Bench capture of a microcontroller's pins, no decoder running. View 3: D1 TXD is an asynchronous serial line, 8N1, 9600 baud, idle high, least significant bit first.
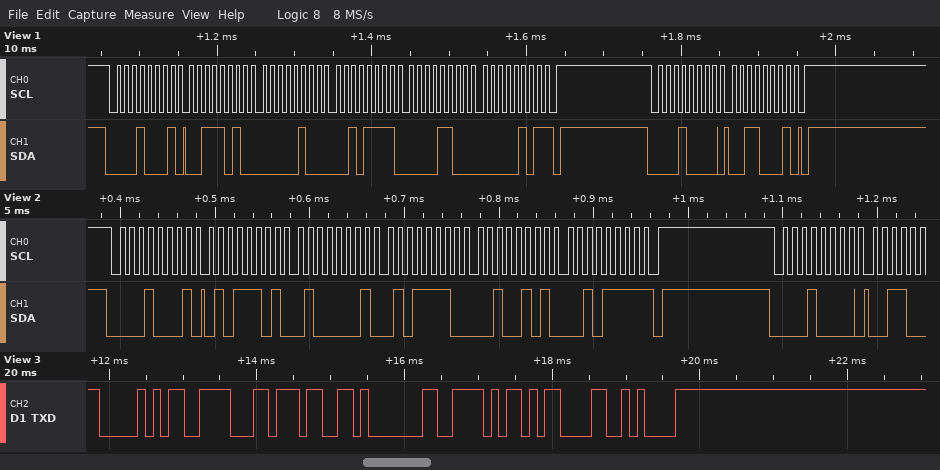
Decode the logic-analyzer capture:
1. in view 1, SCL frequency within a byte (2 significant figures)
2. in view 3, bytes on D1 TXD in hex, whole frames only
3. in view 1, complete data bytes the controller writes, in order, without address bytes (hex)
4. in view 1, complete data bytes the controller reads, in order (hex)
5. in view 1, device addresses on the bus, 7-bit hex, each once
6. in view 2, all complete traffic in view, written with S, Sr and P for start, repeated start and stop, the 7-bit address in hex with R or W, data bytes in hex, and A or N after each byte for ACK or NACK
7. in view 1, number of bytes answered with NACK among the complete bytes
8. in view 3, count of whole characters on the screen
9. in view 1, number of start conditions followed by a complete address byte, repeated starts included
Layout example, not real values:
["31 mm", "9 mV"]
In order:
["100 kHz", "50 1E 37 01 5E 0D 0A", "31", "3A 04 2F 0C 05", "0x08", "S 08R A 5D A 41 A 5E A 25 A 2F N P S 08W A", "1", "7", "2"]
